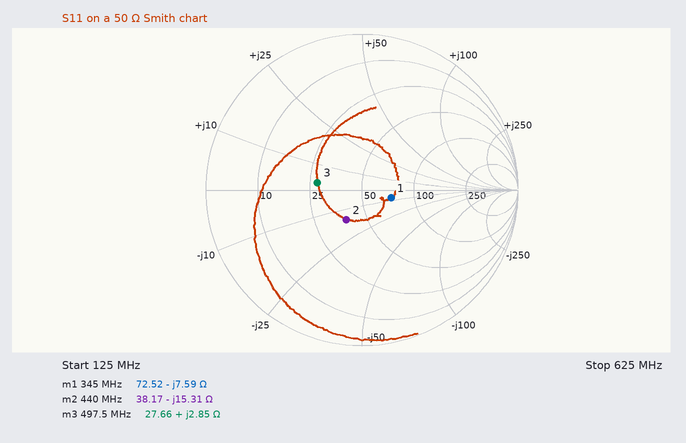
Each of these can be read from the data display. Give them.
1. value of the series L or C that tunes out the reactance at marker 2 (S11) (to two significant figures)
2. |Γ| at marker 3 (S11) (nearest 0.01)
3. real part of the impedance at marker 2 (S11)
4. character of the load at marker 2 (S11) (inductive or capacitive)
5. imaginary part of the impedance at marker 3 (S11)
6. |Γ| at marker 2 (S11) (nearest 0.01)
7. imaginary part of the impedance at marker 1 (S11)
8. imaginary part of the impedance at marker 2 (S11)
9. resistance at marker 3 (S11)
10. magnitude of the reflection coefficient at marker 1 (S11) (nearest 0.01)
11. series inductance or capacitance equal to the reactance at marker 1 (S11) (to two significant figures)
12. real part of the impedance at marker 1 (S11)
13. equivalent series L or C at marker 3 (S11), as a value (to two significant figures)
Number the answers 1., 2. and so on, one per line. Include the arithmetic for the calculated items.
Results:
1. L = 15.31 Ω/(2π × 440 MHz) ≈ 5.5 nH
2. 0.29
3. 38.17 Ω
4. capacitive
5. +2.85 Ω
6. 0.22
7. -7.59 Ω
8. -15.31 Ω
9. 27.66 Ω
10. 0.19
11. C = 1/(2π × 345 MHz × 7.59 Ω) ≈ 61 pF
12. 72.52 Ω
13. L = 2.85 Ω/(2π × 497.5 MHz) ≈ 912 pH, so 910 pH to two significant figures
